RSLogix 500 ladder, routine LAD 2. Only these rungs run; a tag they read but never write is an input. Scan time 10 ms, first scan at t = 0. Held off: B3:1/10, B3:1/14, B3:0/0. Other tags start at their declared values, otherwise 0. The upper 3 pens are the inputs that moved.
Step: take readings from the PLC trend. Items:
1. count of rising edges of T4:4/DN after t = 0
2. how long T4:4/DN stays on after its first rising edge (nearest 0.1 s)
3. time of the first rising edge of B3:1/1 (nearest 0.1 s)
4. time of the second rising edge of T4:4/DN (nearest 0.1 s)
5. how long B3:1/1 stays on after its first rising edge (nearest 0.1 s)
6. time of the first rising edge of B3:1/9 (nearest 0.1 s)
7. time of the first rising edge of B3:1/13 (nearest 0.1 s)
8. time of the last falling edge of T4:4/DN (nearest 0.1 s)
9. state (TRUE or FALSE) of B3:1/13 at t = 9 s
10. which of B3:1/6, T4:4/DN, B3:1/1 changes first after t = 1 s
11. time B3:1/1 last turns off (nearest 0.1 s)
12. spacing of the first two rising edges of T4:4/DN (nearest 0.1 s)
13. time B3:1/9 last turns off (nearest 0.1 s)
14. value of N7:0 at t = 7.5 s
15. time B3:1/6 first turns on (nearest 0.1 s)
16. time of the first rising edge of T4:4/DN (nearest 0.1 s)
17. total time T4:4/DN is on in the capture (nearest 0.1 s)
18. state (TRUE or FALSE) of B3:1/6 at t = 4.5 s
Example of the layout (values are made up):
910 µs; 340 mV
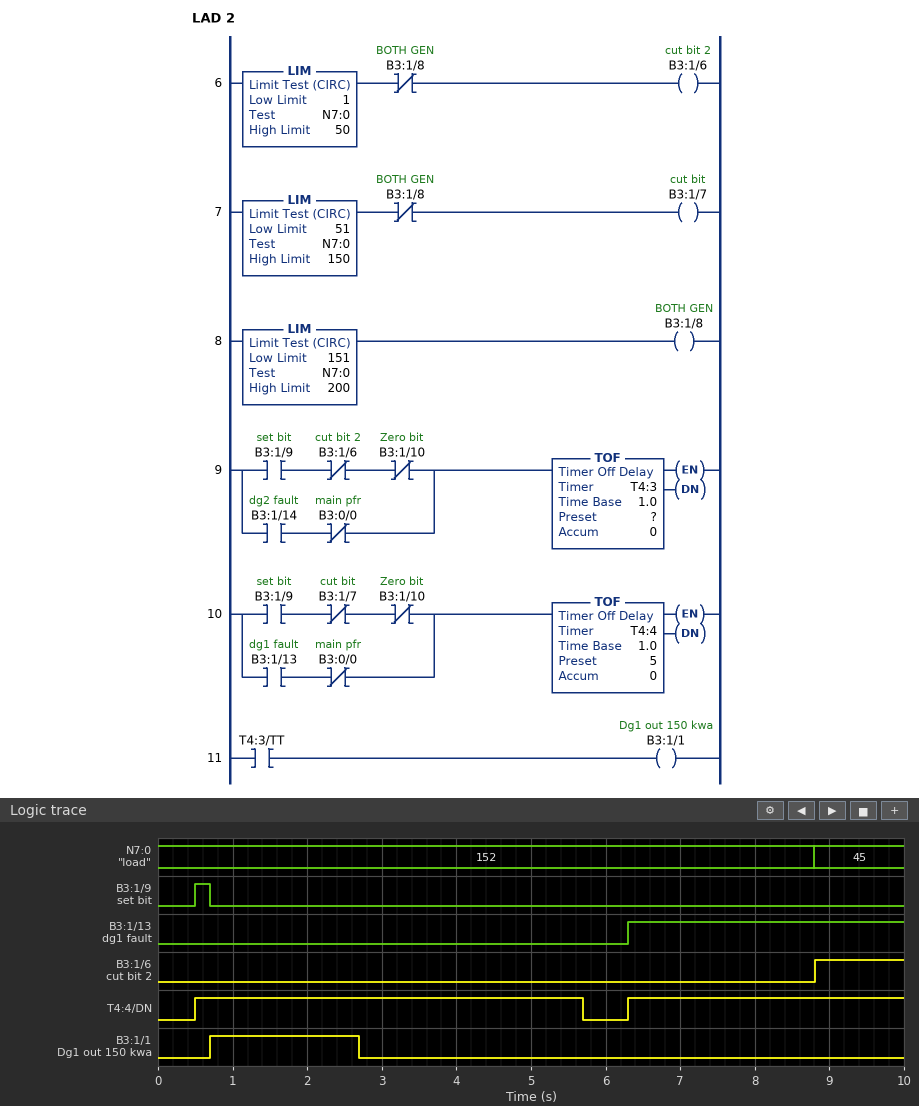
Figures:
2; 5.2 s; 0.7 s; 6.3 s; 2.0 s; 0.5 s; 6.3 s; 5.7 s; TRUE; B3:1/1; 2.7 s; 5.8 s; 0.7 s; 152; 8.8 s; 0.5 s; 8.9 s; FALSE
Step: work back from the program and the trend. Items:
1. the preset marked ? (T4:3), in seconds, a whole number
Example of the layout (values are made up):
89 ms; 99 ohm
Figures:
2 s
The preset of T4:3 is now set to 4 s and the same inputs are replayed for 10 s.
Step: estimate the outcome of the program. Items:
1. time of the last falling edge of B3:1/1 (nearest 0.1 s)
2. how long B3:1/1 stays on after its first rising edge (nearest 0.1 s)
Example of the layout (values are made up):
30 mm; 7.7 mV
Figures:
4.7 s; 4.0 s
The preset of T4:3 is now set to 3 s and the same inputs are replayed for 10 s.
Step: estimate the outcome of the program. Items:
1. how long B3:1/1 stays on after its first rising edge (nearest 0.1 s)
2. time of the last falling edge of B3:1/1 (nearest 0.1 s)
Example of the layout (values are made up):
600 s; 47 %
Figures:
3.0 s; 3.7 s
